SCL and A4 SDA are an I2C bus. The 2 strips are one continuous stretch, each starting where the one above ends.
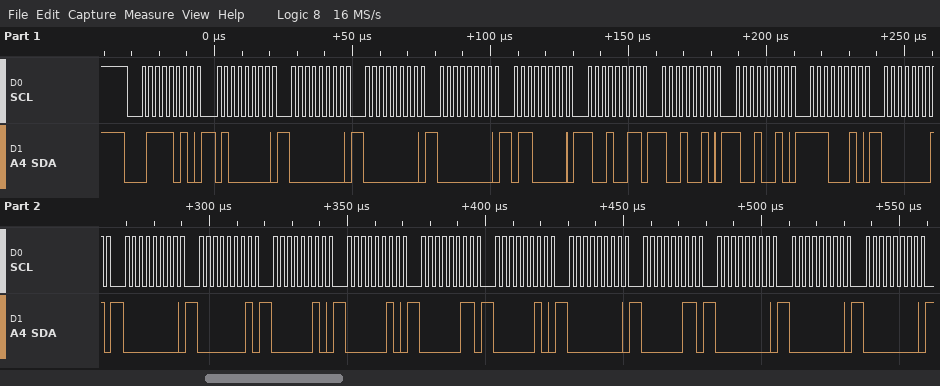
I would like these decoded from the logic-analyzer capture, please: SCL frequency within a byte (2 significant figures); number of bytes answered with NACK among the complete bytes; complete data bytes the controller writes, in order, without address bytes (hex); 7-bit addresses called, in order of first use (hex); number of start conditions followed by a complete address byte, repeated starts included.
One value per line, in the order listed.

400 kHz
0
40 00 00 00 60 93 92 92 E2 01 00 01 02 02 03 02 00 03 00 00 00
0x3D
1
